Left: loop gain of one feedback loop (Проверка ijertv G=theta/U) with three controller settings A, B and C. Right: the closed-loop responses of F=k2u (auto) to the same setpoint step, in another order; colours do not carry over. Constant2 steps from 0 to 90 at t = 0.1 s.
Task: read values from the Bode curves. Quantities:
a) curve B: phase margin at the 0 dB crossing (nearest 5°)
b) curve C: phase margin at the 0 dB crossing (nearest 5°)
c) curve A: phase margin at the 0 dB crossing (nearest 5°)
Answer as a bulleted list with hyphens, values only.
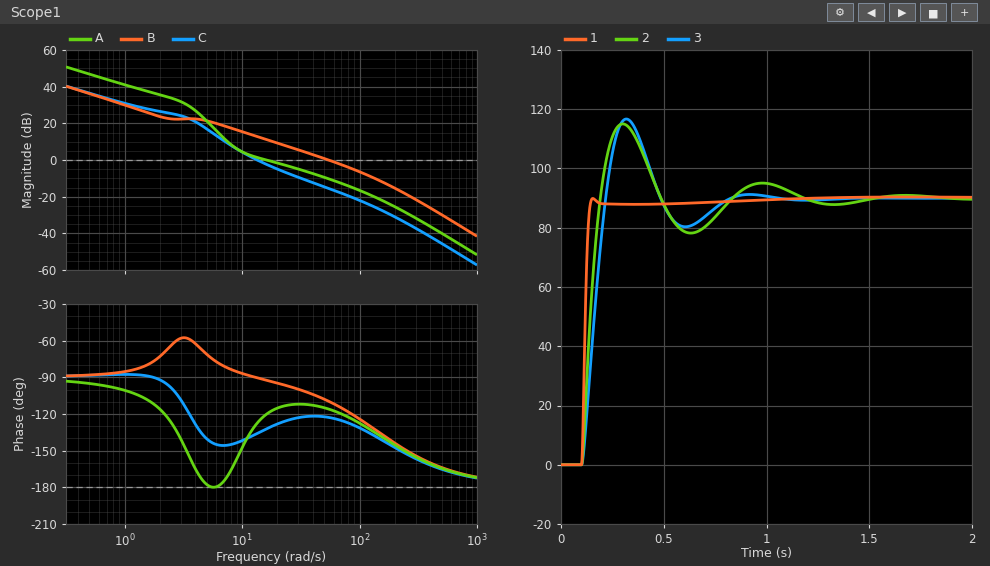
- 70°
- 45°
- 60°
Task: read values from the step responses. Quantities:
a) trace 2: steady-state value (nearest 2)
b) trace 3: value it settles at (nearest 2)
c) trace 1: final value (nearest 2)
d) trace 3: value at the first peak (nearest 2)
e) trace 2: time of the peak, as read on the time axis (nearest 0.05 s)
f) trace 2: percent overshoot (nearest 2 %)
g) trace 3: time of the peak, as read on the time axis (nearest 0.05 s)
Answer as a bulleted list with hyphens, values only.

- 90
- 90
- 90
- 116
- 0.30 s
- 28 %
- 0.30 s
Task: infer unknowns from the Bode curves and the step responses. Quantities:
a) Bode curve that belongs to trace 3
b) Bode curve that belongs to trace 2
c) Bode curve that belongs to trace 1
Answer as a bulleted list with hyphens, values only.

- C
- A
- B
